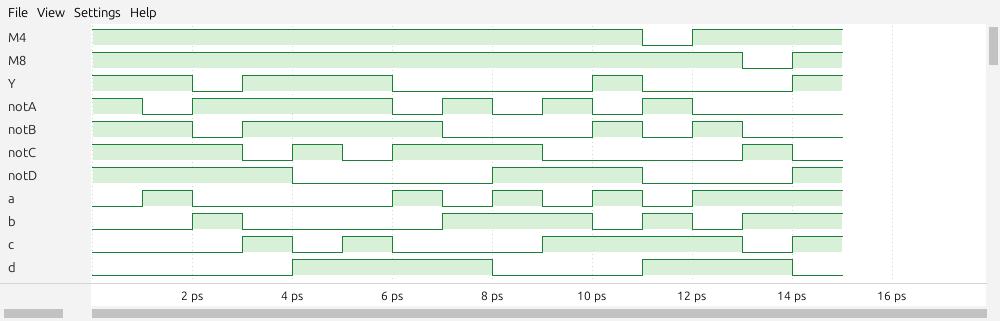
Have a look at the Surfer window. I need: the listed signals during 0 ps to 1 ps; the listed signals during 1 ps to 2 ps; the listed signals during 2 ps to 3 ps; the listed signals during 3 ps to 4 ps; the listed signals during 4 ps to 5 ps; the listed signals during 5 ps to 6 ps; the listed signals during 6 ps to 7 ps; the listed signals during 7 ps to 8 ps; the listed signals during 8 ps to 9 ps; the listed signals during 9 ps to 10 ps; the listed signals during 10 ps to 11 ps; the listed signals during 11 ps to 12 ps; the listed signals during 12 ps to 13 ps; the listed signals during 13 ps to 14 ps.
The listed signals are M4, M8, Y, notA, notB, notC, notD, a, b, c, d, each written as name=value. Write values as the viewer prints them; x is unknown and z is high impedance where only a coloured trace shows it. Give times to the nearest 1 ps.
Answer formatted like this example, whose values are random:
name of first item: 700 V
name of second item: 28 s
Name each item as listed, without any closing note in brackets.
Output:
the listed signals during 0 ps to 1 ps: M4=1, M8=1, Y=1, notA=1, notB=1, notC=1, notD=1, a=0, b=0, c=0, d=0
the listed signals during 1 ps to 2 ps: M4=1, M8=1, Y=1, notA=0, notB=1, notC=1, notD=1, a=1, b=0, c=0, d=0
the listed signals during 2 ps to 3 ps: M4=1, M8=1, Y=0, notA=1, notB=0, notC=1, notD=1, a=0, b=1, c=0, d=0
the listed signals during 3 ps to 4 ps: M4=1, M8=1, Y=1, notA=1, notB=1, notC=0, notD=1, a=0, b=0, c=1, d=0
the listed signals during 4 ps to 5 ps: M4=1, M8=1, Y=1, notA=1, notB=1, notC=1, notD=0, a=0, b=0, c=0, d=1
the listed signals during 5 ps to 6 ps: M4=1, M8=1, Y=1, notA=1, notB=1, notC=0, notD=0, a=0, b=0, c=1, d=1
the listed signals during 6 ps to 7 ps: M4=1, M8=1, Y=0, notA=0, notB=1, notC=1, notD=0, a=1, b=0, c=0, d=1
the listed signals during 7 ps to 8 ps: M4=1, M8=1, Y=0, notA=1, notB=0, notC=1, notD=0, a=0, b=1, c=0, d=1
the listed signals during 8 ps to 9 ps: M4=1, M8=1, Y=0, notA=0, notB=0, notC=1, notD=1, a=1, b=1, c=0, d=0
the listed signals during 9 ps to 10 ps: M4=1, M8=1, Y=0, notA=1, notB=0, notC=0, notD=1, a=0, b=1, c=1, d=0
the listed signals during 10 ps to 11 ps: M4=1, M8=1, Y=1, notA=0, notB=1, notC=0, notD=1, a=1, b=0, c=1, d=0
the listed signals during 11 ps to 12 ps: M4=0, M8=1, Y=0, notA=1, notB=0, notC=0, notD=0, a=0, b=1, c=1, d=1
the listed signals during 12 ps to 13 ps: M4=1, M8=1, Y=0, notA=0, notB=1, notC=0, notD=0, a=1, b=0, c=1, d=1
the listed signals during 13 ps to 14 ps: M4=1, M8=0, Y=0, notA=0, notB=0, notC=1, notD=0, a=1, b=1, c=0, d=1
